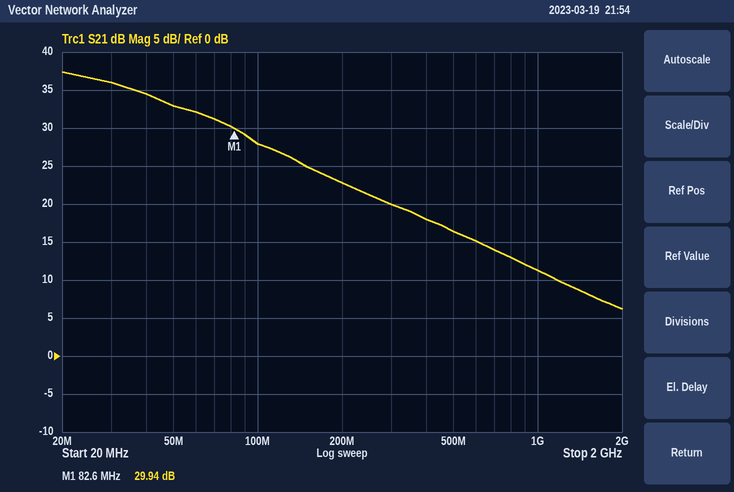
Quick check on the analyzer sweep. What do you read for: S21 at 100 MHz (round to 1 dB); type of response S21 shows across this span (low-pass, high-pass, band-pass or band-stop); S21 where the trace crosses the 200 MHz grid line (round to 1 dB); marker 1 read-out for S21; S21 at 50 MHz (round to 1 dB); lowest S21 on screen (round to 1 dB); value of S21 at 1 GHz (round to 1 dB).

28 dB
low-pass
23 dB
29.94 dB
33 dB
6 dB
11 dB
